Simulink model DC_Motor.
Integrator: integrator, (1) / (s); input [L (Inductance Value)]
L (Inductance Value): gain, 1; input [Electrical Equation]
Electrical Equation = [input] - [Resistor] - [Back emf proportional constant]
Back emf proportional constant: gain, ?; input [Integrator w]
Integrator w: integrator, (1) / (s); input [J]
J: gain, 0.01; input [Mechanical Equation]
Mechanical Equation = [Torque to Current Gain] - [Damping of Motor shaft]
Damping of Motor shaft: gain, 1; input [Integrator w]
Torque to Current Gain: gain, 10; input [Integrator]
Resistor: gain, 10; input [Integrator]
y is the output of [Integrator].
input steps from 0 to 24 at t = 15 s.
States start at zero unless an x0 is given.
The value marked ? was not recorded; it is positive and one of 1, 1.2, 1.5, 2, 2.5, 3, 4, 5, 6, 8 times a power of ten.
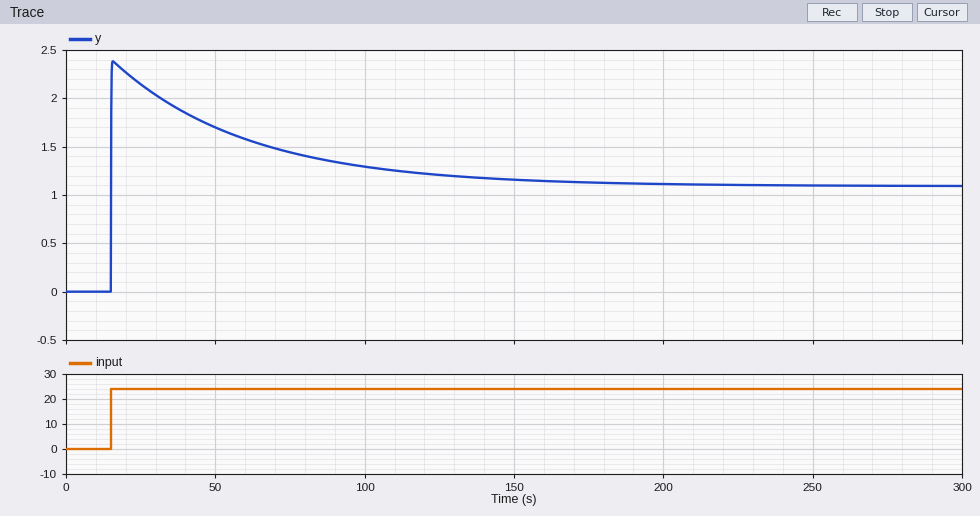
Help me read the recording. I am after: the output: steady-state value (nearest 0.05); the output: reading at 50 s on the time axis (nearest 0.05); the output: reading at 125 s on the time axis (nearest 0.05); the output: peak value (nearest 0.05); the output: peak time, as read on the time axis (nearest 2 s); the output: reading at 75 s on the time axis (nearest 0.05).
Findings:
1.10
1.70
1.20
2.40
16 s
1.45
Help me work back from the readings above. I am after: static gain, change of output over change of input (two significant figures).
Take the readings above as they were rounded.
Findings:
0.046
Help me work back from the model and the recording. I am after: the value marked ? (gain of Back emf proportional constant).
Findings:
1.2
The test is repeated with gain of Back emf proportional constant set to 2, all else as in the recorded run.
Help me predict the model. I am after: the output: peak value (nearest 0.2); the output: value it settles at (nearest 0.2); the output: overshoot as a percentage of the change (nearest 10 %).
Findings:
2.4
0.8
200 %
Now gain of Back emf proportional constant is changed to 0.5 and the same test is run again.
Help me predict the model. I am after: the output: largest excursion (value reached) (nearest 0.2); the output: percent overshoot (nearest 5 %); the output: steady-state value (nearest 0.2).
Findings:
2.4
50 %
1.6
